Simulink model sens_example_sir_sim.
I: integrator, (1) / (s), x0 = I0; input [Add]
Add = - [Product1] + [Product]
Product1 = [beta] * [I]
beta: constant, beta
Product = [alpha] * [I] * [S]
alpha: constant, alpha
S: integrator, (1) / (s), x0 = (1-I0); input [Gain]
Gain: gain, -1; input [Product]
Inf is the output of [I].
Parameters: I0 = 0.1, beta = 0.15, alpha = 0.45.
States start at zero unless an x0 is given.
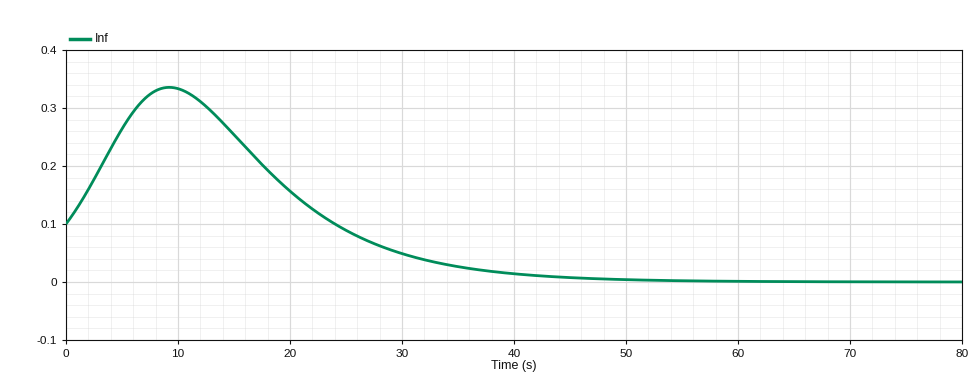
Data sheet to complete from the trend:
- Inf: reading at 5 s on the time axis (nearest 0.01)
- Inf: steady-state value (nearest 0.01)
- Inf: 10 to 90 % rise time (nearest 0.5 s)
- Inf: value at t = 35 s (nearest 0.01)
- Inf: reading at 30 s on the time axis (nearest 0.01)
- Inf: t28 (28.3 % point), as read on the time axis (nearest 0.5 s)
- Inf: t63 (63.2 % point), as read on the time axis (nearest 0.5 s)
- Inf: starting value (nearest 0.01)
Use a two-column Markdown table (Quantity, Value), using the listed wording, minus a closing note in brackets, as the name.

| Quantity | Value |
|---|---|
| Inf: reading at 5 s on the time axis | 0.26 |
| Inf: steady-state value | 0.00 |
| Inf: 10 to 90 % rise time | 18.0 s |
| Inf: value at t = 35 s | 0.03 |
| Inf: reading at 30 s on the time axis | 0.05 |
| Inf: t28 (28.3 % point), as read on the time axis | 27.0 s |
| Inf: t63 (63.2 % point), as read on the time axis | 32.5 s |
| Inf: starting value | 0.10 |
